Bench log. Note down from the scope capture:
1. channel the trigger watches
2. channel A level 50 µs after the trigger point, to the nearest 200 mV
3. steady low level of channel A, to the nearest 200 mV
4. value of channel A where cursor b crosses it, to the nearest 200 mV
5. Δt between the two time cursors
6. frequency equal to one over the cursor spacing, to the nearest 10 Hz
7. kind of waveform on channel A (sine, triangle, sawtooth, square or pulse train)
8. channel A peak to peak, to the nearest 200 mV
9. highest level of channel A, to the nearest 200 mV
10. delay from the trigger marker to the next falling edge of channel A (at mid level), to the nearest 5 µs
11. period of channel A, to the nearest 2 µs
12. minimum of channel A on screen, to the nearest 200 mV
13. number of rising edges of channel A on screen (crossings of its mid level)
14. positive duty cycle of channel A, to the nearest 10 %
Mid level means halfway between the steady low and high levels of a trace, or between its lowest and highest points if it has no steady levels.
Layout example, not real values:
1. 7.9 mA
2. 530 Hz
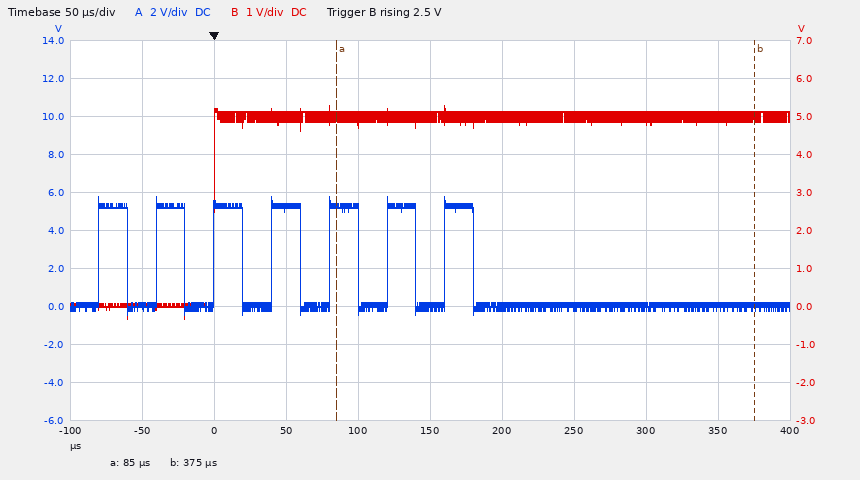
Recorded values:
1. channel B
2. 5.2 V
3. 0.0 V
4. 0.0 V
5. 290 µs
6. 3.45 kHz
7. square
8. 6.2 V
9. 5.8 V
10. 20 µs
11. 40 µs
12. -400 mV
13. 7
14. 50 %
